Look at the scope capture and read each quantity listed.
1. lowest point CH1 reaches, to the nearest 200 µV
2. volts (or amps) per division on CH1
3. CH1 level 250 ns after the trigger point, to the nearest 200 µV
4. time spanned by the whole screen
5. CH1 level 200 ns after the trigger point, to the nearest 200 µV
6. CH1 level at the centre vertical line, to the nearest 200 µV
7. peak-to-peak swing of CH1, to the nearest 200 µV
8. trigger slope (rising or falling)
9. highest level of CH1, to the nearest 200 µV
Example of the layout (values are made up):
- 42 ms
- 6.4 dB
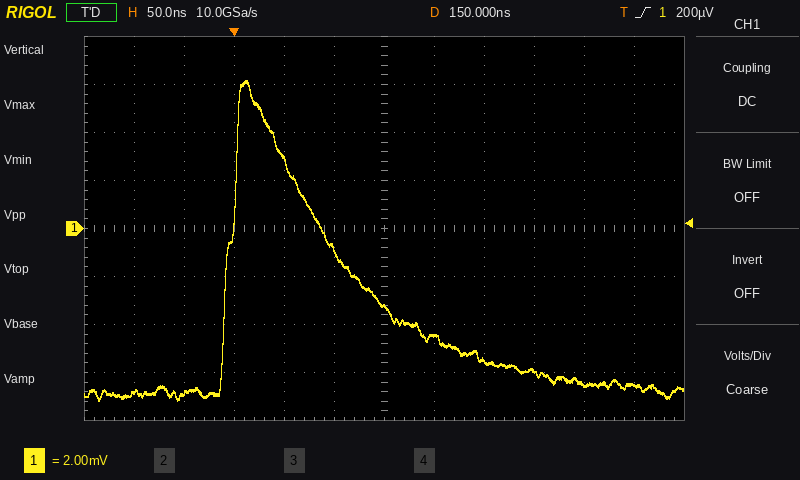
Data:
- -7.2 mV
- 2 mV
- -5.6 mV
- 600 ns
- -4.4 mV
- -3.2 mV
- 13.4 mV
- rising
- 6.2 mV
